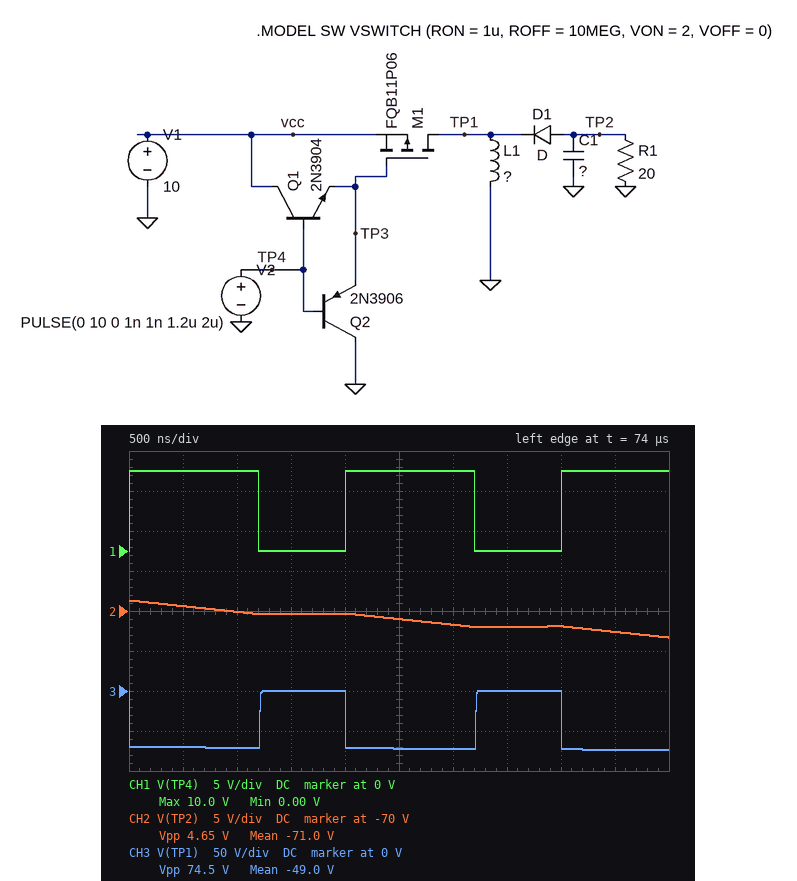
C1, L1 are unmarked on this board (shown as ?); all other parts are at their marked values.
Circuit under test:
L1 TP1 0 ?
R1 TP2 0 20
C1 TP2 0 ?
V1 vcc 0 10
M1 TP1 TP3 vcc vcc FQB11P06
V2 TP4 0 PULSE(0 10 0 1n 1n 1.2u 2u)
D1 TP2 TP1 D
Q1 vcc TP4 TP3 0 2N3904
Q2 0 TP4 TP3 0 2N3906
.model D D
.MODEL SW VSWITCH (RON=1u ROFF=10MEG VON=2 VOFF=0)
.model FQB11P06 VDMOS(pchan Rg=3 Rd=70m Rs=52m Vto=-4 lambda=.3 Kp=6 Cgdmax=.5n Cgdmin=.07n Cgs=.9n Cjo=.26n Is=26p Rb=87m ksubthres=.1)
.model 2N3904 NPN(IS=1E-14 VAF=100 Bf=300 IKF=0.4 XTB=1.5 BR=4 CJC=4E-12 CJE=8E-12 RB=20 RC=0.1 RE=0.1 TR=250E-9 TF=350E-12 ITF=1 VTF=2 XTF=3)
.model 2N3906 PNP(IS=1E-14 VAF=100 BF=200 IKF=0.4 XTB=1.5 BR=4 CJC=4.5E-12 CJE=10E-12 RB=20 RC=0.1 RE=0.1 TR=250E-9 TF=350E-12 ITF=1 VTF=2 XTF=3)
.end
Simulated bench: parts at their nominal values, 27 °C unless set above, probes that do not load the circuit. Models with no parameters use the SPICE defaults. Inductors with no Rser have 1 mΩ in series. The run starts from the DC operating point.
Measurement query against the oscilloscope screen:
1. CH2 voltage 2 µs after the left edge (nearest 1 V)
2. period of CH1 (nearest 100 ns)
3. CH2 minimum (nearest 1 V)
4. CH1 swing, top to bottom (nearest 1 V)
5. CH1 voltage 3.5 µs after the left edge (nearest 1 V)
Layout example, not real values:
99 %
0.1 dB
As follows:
-70 V
2.0 µs
-73 V
10 V
0 V
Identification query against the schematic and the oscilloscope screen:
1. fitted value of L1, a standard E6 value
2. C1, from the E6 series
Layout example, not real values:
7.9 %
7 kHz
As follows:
330 µH
33 µF
